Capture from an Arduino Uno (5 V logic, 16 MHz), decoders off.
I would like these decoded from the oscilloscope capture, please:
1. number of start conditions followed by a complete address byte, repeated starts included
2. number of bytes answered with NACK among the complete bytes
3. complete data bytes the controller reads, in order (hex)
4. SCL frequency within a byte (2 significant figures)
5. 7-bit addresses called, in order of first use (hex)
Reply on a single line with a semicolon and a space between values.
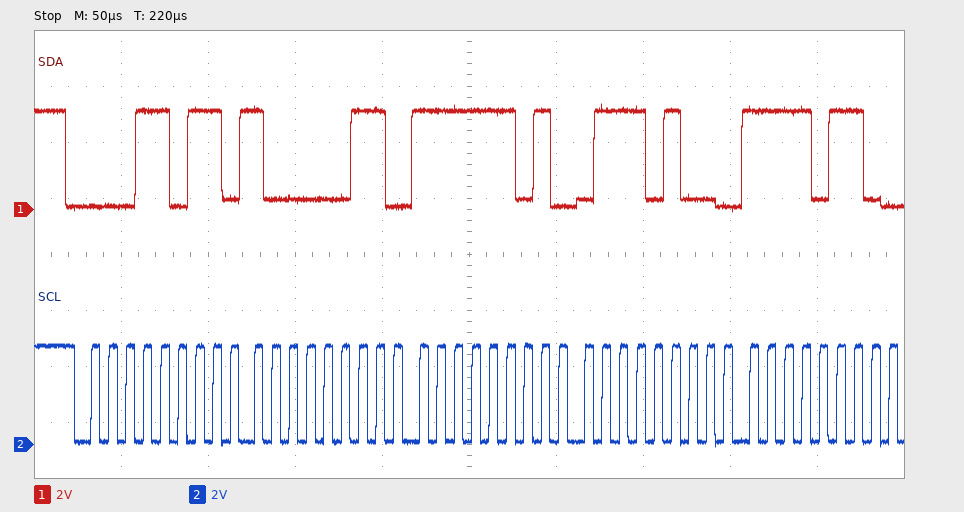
1; 0; 83 FD 74 F6; 100 kHz; 0x0D
